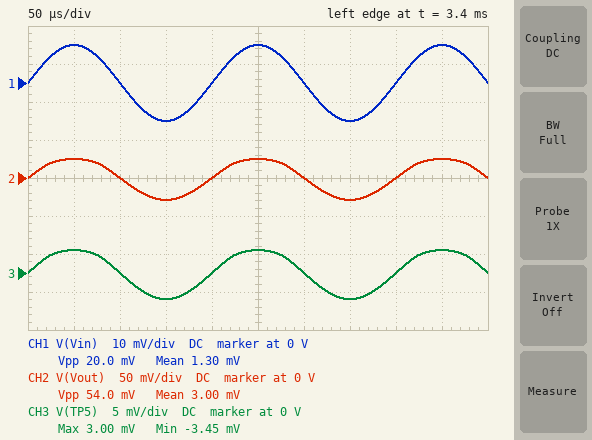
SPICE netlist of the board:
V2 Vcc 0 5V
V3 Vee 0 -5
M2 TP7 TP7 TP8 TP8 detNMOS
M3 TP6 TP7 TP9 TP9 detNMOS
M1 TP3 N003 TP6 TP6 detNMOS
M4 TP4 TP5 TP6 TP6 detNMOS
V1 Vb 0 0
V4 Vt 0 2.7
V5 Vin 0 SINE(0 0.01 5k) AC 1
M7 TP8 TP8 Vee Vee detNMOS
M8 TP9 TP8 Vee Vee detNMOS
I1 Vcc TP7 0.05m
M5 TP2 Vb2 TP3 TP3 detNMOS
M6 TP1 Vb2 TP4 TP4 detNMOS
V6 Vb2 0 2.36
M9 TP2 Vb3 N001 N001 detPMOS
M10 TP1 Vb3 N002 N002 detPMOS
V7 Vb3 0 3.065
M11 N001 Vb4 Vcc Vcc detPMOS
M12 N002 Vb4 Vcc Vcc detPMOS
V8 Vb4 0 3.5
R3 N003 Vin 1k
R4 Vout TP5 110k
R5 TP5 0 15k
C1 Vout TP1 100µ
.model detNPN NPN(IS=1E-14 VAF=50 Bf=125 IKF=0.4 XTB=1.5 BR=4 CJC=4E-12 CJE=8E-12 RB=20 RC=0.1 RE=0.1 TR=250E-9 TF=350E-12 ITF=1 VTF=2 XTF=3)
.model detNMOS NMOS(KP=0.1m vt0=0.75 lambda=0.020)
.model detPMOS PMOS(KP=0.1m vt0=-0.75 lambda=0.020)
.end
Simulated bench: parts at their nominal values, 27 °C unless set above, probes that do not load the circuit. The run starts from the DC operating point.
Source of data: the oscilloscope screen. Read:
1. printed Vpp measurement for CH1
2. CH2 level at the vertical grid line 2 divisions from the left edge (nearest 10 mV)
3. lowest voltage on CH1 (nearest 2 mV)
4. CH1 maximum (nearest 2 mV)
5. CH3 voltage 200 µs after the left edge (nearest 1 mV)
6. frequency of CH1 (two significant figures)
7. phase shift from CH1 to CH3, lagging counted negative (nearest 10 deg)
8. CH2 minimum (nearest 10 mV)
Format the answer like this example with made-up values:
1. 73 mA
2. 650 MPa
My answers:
1. 20.0 mV
2. 0 V
3. -10 mV
4. 10 mV
5. 0 V
6. 5.0 kHz
7. 0 deg
8. -30 mV
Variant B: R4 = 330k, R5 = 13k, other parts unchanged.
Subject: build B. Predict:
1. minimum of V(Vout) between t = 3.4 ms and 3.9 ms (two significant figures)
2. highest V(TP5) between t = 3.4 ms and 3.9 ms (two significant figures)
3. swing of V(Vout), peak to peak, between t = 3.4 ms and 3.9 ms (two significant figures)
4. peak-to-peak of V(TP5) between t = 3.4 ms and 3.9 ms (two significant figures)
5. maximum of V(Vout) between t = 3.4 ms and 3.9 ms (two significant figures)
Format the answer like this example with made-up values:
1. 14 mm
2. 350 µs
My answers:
1. -81 mV
2. 2.6 mV
3. 150 mV
4. 5.7 mV
5. 69 mV
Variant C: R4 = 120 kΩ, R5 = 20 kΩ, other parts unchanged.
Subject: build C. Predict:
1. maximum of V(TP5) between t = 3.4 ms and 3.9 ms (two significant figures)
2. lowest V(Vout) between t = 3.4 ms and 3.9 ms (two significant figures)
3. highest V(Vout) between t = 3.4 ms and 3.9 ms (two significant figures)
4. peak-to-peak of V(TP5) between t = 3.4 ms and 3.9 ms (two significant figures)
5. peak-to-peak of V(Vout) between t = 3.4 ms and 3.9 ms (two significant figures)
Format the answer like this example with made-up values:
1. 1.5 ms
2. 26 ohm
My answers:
1. 3.8 mV
2. -29 mV
3. 26 mV
4. 7.9 mV
5. 55 mV
